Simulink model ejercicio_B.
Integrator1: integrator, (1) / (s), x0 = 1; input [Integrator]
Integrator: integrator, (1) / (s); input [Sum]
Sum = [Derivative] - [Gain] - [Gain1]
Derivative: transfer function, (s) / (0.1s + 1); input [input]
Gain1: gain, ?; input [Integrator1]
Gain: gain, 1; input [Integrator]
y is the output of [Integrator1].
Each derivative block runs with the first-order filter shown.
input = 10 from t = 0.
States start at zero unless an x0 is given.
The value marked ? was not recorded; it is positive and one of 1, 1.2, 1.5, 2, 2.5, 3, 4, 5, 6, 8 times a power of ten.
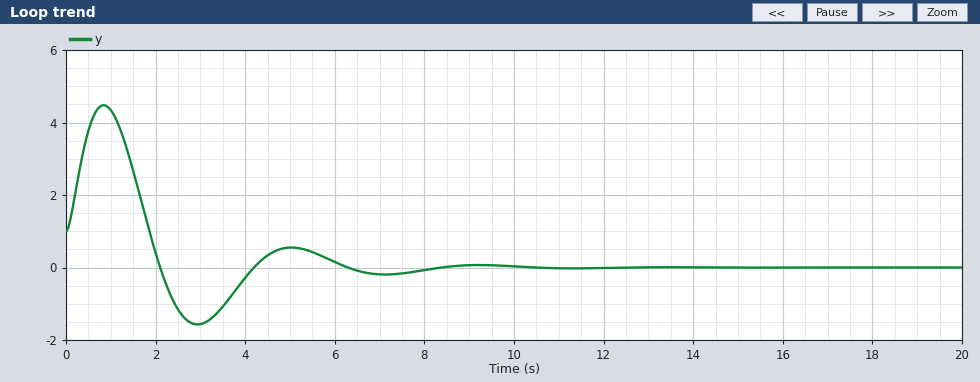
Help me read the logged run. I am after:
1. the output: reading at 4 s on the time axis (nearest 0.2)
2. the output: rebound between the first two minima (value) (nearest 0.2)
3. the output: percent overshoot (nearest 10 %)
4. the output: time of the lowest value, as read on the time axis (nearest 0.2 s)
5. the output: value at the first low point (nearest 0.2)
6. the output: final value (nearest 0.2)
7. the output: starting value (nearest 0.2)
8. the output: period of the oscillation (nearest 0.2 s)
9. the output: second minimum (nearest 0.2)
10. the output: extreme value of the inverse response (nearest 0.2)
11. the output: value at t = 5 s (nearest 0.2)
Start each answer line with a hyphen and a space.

- -0.2
- 0.6
- 160 %
- 3.0 s
- -1.6
- 0.0
- 1.0
- 4.2 s
- -0.2
- 4.4
- 0.6
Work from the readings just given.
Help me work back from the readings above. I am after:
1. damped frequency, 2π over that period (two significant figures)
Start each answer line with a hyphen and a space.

- 1.5 rad/s
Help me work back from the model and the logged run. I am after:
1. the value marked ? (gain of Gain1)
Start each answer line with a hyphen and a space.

- 2.5
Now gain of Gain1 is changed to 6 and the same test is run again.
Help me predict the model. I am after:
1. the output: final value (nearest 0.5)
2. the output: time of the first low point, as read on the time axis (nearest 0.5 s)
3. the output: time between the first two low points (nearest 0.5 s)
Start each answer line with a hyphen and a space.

- 0.0
- 2.0 s
- 2.5 s
